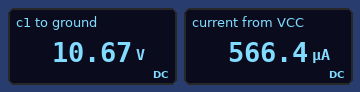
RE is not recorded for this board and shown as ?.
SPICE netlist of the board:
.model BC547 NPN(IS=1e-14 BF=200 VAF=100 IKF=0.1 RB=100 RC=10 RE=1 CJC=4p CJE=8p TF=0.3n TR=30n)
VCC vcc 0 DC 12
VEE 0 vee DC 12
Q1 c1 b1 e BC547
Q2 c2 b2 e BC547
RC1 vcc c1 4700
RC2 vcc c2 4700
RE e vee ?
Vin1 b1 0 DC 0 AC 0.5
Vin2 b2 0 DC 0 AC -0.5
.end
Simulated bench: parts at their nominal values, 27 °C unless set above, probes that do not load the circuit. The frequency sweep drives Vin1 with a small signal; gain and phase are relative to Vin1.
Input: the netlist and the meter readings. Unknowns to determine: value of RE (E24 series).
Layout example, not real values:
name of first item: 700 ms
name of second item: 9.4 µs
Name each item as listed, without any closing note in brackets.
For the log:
value of RE: 20 kΩ
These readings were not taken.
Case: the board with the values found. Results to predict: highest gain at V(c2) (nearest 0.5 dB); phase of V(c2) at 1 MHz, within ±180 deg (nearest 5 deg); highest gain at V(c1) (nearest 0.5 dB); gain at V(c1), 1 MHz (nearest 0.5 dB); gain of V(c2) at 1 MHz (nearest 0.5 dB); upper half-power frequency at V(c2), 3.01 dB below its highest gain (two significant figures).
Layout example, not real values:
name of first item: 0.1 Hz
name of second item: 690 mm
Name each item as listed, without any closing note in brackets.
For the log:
highest gain at V(c2): 31.5 dB
phase of V(c2) at 1 MHz, within ±180 deg: -5 deg
highest gain at V(c1): 31.5 dB
gain at V(c1), 1 MHz: 31.5 dB
gain of V(c2) at 1 MHz: 31.5 dB
upper half-power frequency at V(c2), 3.01 dB below its highest gain: 9.5 MHz
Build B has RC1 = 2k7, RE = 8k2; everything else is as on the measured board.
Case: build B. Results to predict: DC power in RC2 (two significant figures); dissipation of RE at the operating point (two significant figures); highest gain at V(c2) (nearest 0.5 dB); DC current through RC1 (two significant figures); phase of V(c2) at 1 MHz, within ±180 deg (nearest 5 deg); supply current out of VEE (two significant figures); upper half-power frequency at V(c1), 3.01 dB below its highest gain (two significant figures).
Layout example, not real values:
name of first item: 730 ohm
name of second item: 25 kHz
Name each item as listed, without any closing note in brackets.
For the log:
DC power in RC2: 2.2 mW
dissipation of RE at the operating point: 16 mW
highest gain at V(c2): 39.0 dB
DC current through RC1: 690 µA
phase of V(c2) at 1 MHz, within ±180 deg: -10 deg
supply current out of VEE: 1.4 mA
upper half-power frequency at V(c1), 3.01 dB below its highest gain: 7.0 MHz
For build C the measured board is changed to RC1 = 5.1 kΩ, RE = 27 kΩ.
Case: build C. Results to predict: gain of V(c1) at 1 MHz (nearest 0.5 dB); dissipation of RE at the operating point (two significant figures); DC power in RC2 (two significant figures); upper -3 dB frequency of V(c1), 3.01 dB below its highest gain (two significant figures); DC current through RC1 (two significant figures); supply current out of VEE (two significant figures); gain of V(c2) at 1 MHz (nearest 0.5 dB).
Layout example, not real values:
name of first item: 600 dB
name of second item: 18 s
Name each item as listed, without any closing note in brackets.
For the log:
gain of V(c1) at 1 MHz: 29.5 dB
dissipation of RE at the operating point: 4.8 mW
DC power in RC2: 210 µW
upper -3 dB frequency of V(c1), 3.01 dB below its highest gain: 10 MHz
DC current through RC1: 210 µA
supply current out of VEE: 420 µA
gain of V(c2) at 1 MHz: 29.0 dB
